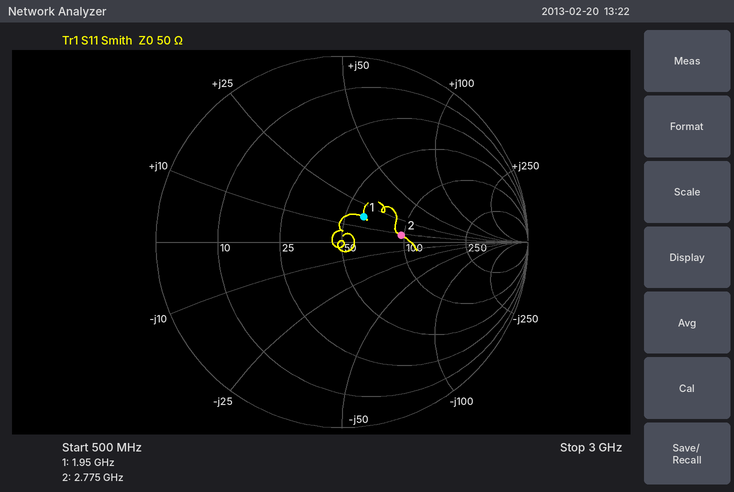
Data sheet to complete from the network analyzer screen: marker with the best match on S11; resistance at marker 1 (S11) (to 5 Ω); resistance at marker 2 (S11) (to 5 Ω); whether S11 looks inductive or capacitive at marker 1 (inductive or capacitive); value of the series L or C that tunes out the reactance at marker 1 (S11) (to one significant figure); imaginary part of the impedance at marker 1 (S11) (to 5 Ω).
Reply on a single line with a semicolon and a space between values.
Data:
marker 1; 60 Ω; 95 Ω; inductive; 5 pF; +15 Ω
